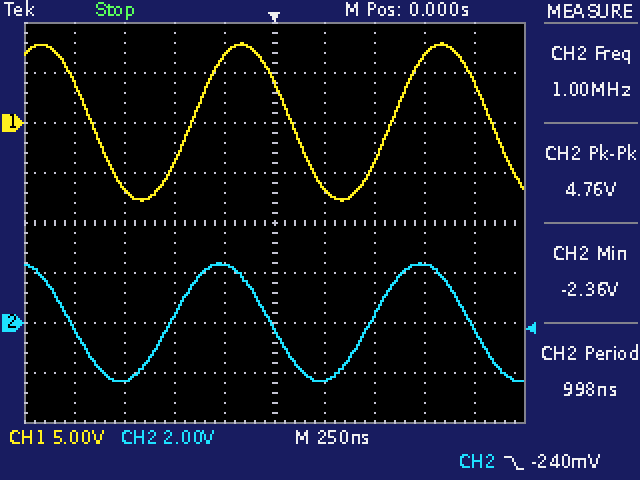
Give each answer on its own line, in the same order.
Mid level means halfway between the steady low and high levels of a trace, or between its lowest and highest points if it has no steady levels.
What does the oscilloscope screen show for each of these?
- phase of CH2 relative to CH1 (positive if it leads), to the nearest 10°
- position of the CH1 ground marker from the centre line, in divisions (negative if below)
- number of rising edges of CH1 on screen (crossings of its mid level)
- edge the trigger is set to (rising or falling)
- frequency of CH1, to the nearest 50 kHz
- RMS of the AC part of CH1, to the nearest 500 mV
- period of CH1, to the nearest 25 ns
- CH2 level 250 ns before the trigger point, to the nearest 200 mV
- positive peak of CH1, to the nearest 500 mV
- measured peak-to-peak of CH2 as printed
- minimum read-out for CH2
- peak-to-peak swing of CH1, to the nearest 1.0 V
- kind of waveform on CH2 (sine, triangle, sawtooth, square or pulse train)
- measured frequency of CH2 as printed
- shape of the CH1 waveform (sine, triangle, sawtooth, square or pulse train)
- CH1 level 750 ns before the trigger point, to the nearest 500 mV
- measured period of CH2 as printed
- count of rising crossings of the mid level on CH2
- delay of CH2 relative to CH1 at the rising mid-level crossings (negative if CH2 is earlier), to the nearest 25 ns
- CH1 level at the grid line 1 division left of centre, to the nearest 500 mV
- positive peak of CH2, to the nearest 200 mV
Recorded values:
+40°
+2.0 div
2
falling
1.00 MHz
5.5 V
1.000 µs
2.4 V
8.0 V
4.76 V
-2.36 V
16.0 V
sine
1.00 MHz
sine
-6.5 V
998 ns
2
-100 ns
6.5 V
2.4 V
